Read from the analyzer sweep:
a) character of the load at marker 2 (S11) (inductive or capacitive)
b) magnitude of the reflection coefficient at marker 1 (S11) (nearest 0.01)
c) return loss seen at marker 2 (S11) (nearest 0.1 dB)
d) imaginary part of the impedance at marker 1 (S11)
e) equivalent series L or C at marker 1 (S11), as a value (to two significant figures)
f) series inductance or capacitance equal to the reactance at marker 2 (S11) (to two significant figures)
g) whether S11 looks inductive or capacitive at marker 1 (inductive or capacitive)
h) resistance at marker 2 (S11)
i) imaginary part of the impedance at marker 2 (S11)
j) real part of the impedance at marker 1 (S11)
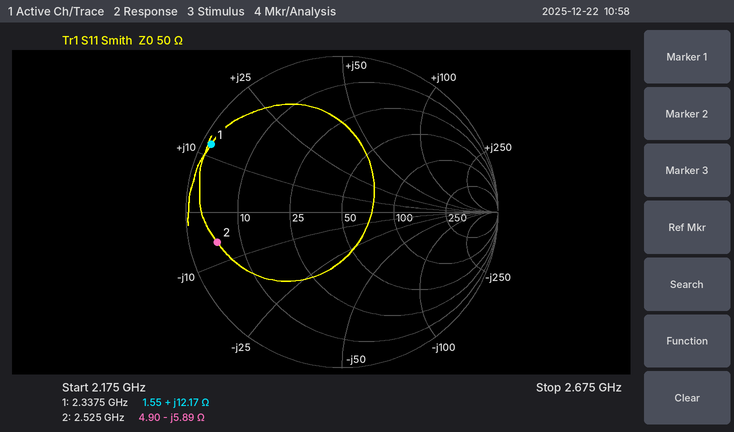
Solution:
capacitive
0.94
1.7 dB
+12.17 Ω
830 pH
11 pF
inductive
4.90 Ω
-5.89 Ω
1.55 Ω
